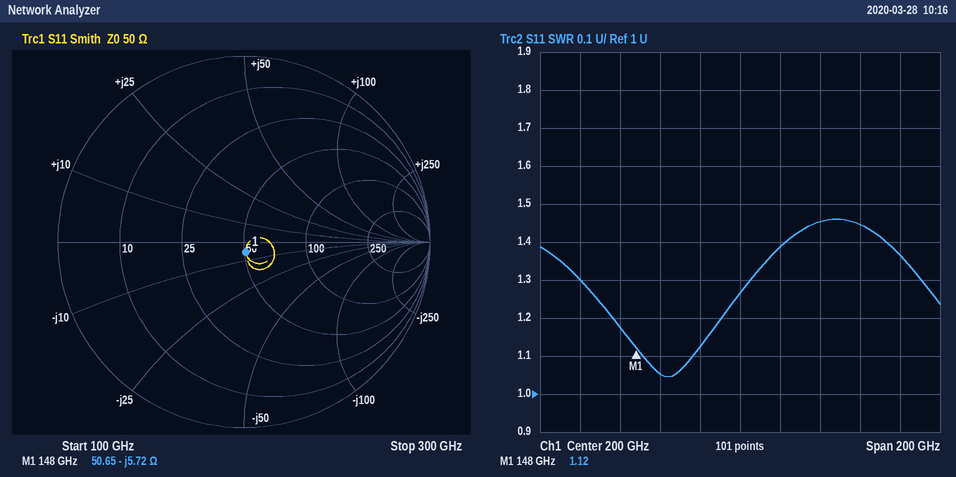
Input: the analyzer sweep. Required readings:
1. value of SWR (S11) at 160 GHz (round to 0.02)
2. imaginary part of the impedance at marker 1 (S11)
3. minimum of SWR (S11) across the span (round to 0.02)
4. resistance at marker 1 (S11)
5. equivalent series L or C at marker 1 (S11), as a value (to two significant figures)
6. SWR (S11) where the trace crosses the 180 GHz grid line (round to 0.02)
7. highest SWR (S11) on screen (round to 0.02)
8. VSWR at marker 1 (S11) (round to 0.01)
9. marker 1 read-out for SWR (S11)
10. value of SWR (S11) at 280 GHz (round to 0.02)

1.06
-5.72 Ω
1.04
50.65 Ω
190 fF
1.12
1.46
1.12
1.12
1.36
